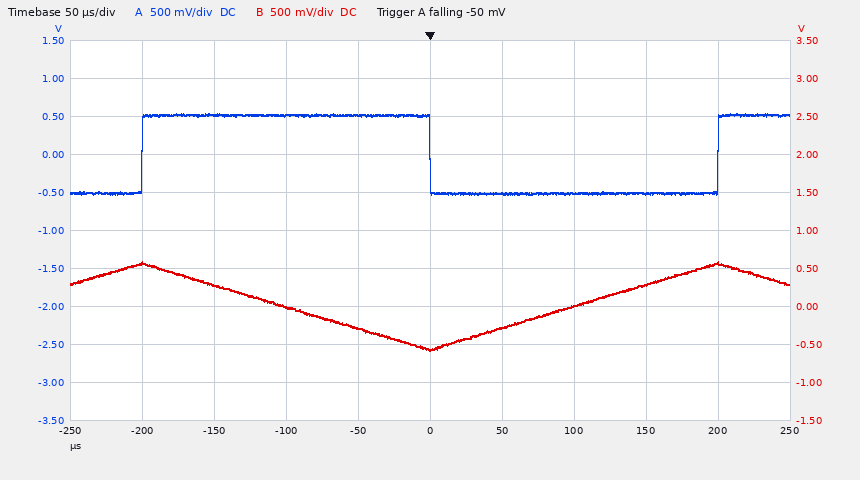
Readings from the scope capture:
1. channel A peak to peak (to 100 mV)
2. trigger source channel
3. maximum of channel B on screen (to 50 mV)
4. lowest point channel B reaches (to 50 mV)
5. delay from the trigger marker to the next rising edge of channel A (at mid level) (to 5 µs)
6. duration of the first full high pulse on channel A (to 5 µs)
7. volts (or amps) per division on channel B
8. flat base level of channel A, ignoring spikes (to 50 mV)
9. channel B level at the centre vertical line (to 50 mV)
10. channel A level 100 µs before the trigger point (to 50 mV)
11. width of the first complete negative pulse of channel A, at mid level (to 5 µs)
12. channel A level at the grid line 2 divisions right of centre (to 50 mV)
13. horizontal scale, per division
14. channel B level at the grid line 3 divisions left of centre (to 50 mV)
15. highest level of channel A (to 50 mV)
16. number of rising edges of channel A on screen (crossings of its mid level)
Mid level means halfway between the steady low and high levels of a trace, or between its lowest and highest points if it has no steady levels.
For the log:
1.10 V
channel A
600 mV
-600 mV
200 µs
200 µs
500 mV
-500 mV
-550 mV
500 mV
200 µs
-500 mV
50 µs
300 mV
550 mV
2
